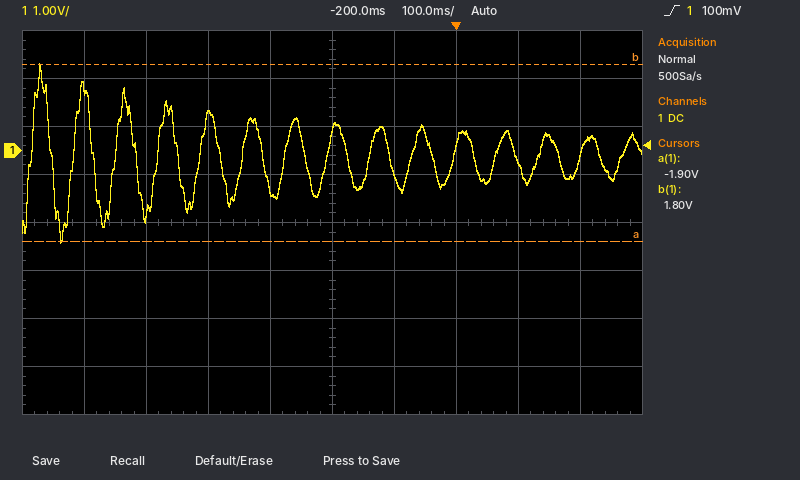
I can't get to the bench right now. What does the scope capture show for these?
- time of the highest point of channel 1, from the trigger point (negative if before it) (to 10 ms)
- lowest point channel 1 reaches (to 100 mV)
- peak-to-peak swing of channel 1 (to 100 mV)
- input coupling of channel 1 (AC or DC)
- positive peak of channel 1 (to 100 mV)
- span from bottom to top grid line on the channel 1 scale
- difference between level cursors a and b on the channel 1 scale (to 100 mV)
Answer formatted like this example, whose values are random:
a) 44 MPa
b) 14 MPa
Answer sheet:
a) -670 ms
b) -1.9 V
c) 3.7 V
d) DC
e) 1.8 V
f) 8 V
g) 3.7 V
